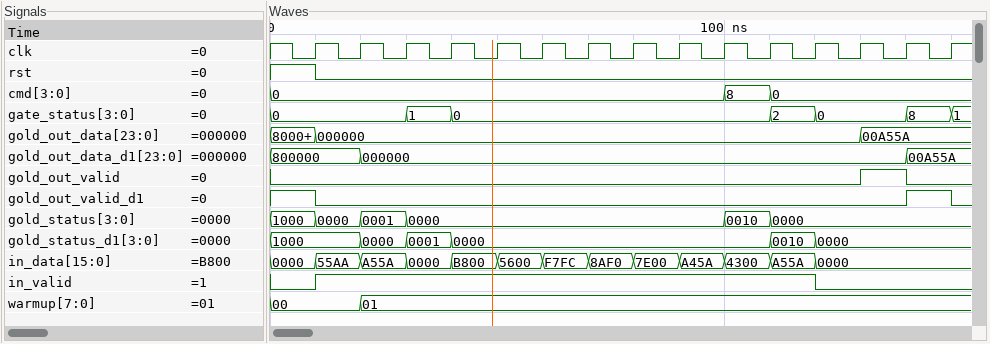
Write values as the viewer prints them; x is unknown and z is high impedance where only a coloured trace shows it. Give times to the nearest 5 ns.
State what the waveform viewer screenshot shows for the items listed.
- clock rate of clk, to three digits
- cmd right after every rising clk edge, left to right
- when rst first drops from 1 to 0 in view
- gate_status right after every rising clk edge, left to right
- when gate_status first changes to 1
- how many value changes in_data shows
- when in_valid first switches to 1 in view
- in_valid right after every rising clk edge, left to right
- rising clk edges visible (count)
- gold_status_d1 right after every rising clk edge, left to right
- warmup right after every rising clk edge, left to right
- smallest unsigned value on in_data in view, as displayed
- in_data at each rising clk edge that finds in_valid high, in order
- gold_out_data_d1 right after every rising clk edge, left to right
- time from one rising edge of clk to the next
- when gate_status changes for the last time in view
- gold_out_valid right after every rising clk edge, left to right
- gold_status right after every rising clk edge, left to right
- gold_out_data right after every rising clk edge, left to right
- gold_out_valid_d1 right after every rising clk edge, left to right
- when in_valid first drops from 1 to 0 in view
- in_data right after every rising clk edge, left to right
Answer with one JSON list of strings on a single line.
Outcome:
["100 MHz", "0, 0, 0, 0, 0, 0, 0, 0, 0, 8, 0, 0, 0, 0, 0", "10 ns", "0, 0, 1, 0, 0, 0, 0, 0, 0, 0, 2, 0, 0, 8, 1", "30 ns", "12", "10 ns", "1 1 1 1 1 1 1 1 1 1 1 0 0 0 0", "15", "1000, 0000, 0001, 0000, 0000, 0000, 0000, 0000, 0000, 0000, 0010, 0000, 0000, 0000, 0000", "00, 01, 01, 01, 01, 01, 01, 01, 01, 01, 01, 01, 01, 01, 01", "0000", "55AA, A55A, 0000, B800, 5600, F7FC, 8AF0, 7E00, A45A, 4300, A55A", "800000, 000000, 000000, 000000, 000000, 000000, 000000, 000000, 000000, 000000, 000000, 000000, 000000, 00A55A, 00A55A", "10 ns", "150 ns", "0 0 0 0 0 0 0 0 0 0 0 0 1 0 0", "0000, 0001, 0000, 0000, 0000, 0000, 0000, 0000, 0000, 0010, 0000, 0000, 0000, 0000, 0000", "000000, 000000, 000000, 000000, 000000, 000000, 000000, 000000, 000000, 000000, 000000, 000000, 00A55A, 00A55A, 00A55A", "0 0 0 0 0 0 0 0 0 0 0 0 0 1 0", "120 ns", "55AA, A55A, 0000, B800, 5600, F7FC, 8AF0, 7E00, A45A, 4300, A55A, 0000, 0000, 0000, 0000"]
